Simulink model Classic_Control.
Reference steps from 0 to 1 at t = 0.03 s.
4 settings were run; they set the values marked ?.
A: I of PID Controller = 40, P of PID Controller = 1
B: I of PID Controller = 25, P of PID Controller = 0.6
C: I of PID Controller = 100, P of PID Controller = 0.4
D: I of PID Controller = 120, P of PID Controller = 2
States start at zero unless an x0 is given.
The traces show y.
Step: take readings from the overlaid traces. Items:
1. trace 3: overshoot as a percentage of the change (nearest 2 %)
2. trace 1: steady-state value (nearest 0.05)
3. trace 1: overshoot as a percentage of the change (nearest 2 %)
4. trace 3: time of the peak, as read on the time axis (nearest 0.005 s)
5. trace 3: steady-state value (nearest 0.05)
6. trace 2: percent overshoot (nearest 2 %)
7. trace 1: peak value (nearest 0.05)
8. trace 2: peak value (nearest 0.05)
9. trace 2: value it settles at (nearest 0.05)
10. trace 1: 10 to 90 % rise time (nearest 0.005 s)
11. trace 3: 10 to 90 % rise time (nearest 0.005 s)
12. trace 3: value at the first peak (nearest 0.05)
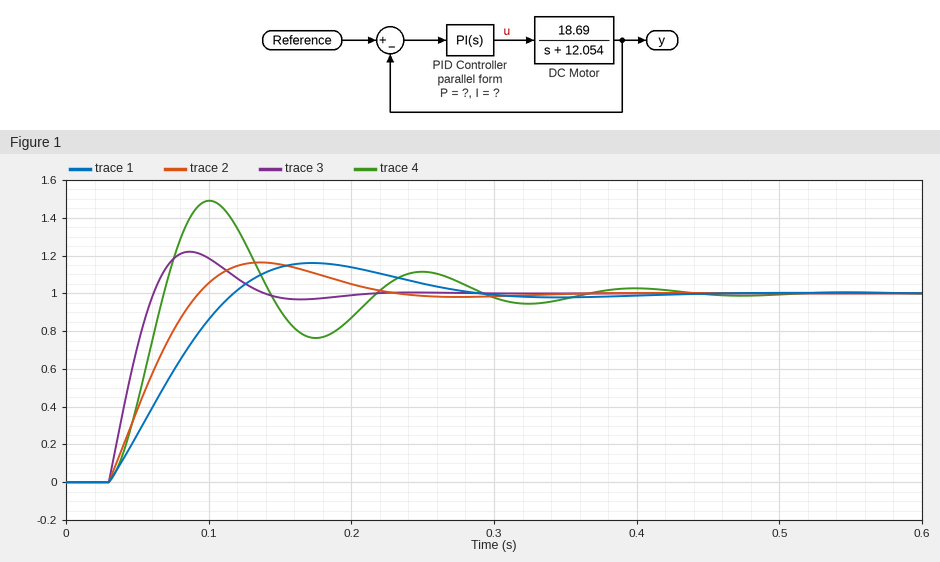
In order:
22 %
1.00
16 %
0.085 s
1.00
16 %
1.15
1.15
1.00
0.065 s
0.025 s
1.20
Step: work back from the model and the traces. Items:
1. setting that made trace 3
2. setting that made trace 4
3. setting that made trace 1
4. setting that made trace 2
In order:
D
C
B
A
